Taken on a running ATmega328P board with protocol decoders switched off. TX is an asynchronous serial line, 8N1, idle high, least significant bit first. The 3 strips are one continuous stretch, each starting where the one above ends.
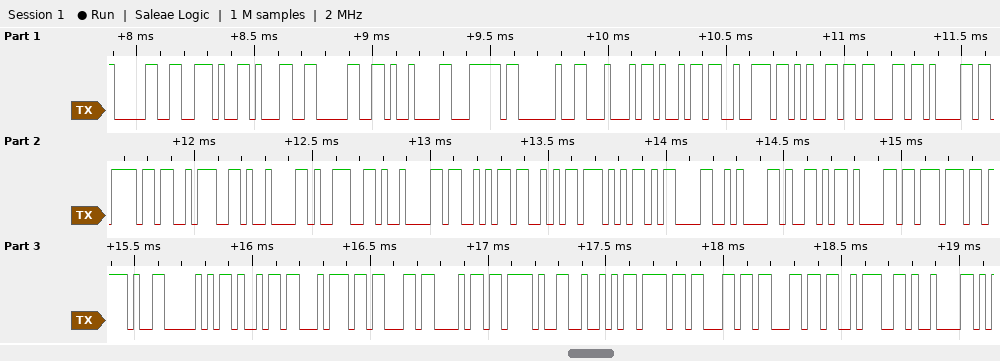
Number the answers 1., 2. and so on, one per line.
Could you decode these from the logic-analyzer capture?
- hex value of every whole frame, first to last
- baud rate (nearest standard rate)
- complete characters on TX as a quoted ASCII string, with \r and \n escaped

1. 30 2E 31 30 09 7C 20 44 69 72 65 63 61 6F 3A 09 39 09 53 53 57 0D 0A 59 61 77 2F 50 69 74 63 68 2F 52 6F 6C 6C 3A 09
2. 38400 baud
3. "0.10\t| Direcao:\t9\tSSW\r\nYaw/Pitch/Roll:\t"
